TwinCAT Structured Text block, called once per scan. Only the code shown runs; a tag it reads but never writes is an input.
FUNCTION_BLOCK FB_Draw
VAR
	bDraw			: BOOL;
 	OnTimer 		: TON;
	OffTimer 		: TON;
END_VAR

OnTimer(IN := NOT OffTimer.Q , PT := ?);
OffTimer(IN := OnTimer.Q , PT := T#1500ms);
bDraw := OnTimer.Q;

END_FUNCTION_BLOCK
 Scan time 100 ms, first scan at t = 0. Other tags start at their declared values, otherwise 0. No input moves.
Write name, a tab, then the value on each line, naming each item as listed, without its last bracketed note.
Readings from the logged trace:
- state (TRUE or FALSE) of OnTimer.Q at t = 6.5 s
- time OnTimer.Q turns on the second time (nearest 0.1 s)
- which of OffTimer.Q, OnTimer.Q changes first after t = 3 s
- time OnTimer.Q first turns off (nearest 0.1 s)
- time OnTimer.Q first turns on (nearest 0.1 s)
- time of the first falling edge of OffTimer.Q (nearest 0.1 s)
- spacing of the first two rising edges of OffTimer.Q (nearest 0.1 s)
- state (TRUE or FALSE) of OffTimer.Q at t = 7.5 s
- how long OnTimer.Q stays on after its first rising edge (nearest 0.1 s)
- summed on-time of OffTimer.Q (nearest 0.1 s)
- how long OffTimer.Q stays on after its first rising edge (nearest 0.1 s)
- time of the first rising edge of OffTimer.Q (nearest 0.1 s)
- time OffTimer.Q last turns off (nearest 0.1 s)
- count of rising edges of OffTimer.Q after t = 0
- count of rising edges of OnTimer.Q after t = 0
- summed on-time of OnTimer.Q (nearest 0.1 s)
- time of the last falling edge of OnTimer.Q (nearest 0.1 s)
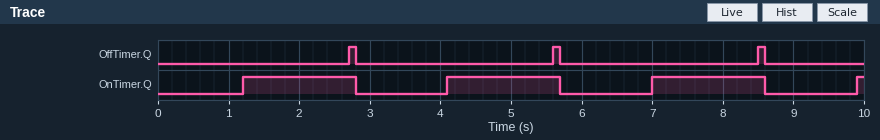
state (TRUE or FALSE) of OnTimer.Q at t = 6.5 s	FALSE
time OnTimer.Q turns on the second time	4.1 s
which of OffTimer.Q, OnTimer.Q changes first after t = 3 s	OnTimer.Q
time OnTimer.Q first turns off	2.8 s
time OnTimer.Q first turns on	1.2 s
time of the first falling edge of OffTimer.Q	2.8 s
spacing of the first two rising edges of OffTimer.Q	2.9 s
state (TRUE or FALSE) of OffTimer.Q at t = 7.5 s	FALSE
how long OnTimer.Q stays on after its first rising edge	1.6 s
summed on-time of OffTimer.Q	0.3 s
how long OffTimer.Q stays on after its first rising edge	0.1 s
time of the first rising edge of OffTimer.Q	2.7 s
time OffTimer.Q last turns off	8.6 s
count of rising edges of OffTimer.Q after t = 0	3
count of rising edges of OnTimer.Q after t = 0	4
summed on-time of OnTimer.Q	4.9 s
time of the last falling edge of OnTimer.Q	8.6 s
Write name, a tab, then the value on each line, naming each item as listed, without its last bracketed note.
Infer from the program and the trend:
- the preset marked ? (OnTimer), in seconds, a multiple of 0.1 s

the preset marked ? (OnTimer), in seconds, a multiple of 0.1 s	1.2 s
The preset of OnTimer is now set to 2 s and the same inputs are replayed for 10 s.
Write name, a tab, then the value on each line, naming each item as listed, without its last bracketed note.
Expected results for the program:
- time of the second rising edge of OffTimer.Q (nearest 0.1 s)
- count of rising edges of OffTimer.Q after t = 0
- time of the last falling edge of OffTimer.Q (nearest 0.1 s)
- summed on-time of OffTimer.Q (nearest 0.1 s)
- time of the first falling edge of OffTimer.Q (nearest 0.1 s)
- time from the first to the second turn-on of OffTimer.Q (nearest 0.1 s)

time of the second rising edge of OffTimer.Q	7.2 s
count of rising edges of OffTimer.Q after t = 0	2
time of the last falling edge of OffTimer.Q	7.3 s
summed on-time of OffTimer.Q	0.2 s
time of the first falling edge of OffTimer.Q	3.6 s
time from the first to the second turn-on of OffTimer.Q	3.7 s
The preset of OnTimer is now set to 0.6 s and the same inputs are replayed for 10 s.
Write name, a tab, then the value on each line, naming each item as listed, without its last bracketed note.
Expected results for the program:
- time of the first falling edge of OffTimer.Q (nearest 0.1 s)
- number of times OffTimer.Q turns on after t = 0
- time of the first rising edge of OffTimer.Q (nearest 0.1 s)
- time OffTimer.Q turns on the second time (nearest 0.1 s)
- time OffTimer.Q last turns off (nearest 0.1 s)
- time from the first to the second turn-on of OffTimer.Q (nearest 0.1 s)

time of the first falling edge of OffTimer.Q	2.2 s
number of times OffTimer.Q turns on after t = 0	4
time of the first rising edge of OffTimer.Q	2.1 s
time OffTimer.Q turns on the second time	4.4 s
time OffTimer.Q last turns off	9.1 s
time from the first to the second turn-on of OffTimer.Q	2.3 s
